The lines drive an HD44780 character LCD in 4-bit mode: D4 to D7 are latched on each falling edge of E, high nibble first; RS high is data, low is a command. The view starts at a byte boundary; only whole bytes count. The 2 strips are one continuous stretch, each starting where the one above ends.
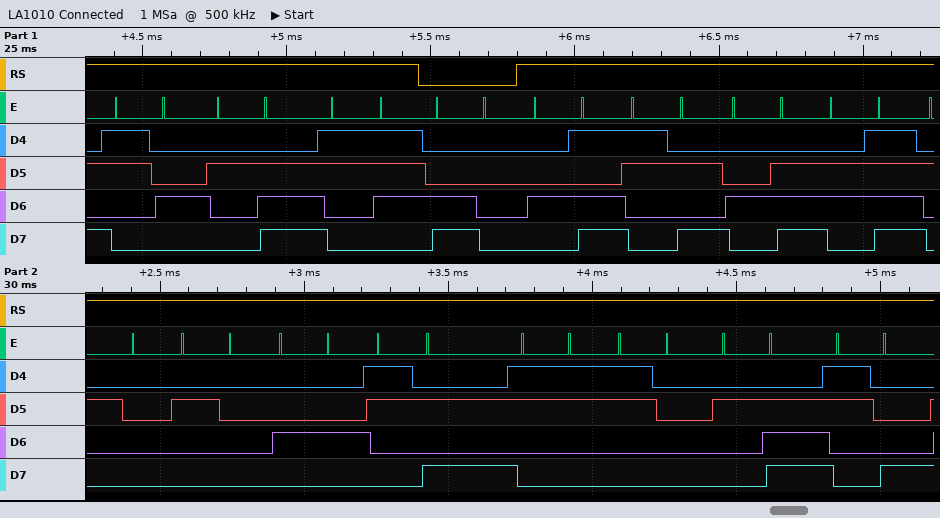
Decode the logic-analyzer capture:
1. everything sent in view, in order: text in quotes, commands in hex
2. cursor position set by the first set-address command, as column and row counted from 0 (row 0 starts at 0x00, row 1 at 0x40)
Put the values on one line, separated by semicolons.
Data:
"4.7" 0xC0 "M:No  D:30.8"; column 0, row 1
